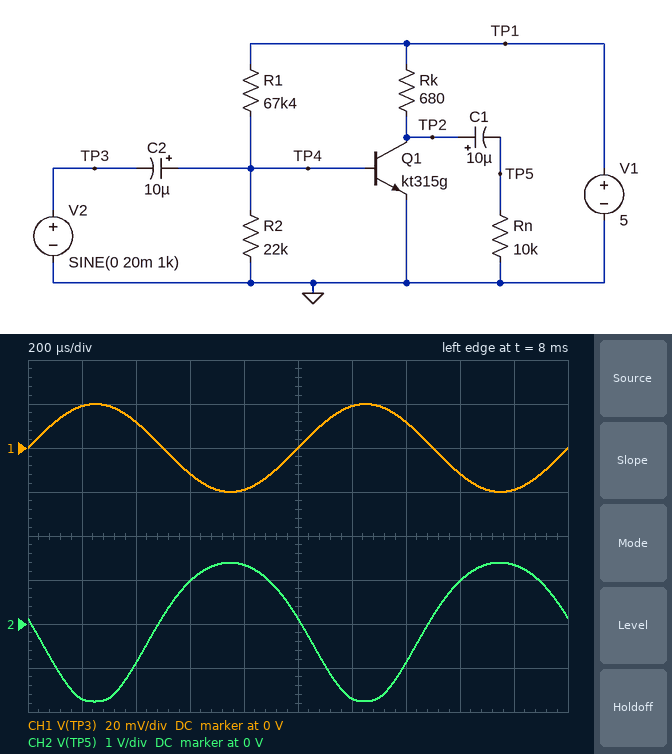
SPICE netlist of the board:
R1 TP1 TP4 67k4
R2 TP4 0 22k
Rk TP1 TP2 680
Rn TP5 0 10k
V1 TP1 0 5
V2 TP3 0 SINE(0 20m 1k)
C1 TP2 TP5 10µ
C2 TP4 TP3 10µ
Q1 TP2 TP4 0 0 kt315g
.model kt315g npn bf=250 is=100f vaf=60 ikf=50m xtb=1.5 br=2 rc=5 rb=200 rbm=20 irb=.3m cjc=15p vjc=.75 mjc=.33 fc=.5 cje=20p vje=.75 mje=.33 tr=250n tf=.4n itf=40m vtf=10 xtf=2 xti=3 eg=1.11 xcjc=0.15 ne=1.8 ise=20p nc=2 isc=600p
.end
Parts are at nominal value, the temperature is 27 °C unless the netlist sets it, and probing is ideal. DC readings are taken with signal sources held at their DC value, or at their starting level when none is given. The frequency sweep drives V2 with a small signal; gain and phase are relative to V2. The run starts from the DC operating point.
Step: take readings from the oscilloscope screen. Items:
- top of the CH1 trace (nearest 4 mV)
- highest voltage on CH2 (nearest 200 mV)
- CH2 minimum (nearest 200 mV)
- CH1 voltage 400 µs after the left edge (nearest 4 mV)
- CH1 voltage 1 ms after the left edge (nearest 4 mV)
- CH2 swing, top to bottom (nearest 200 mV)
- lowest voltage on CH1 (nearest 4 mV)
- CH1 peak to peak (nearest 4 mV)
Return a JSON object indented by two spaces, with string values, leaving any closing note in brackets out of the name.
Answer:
{
  "top of the CH1 trace": "20 mV",
  "highest voltage on CH2": "1.4 V",
  "CH2 minimum": "-1.8 V",
  "CH1 voltage 400 µs after the left edge": "12 mV",
  "CH1 voltage 1 ms after the left edge": "0 V",
  "CH2 swing, top to bottom": "3.2 V",
  "lowest voltage on CH1": "-20 mV",
  "CH1 peak to peak": "40 mV"
}
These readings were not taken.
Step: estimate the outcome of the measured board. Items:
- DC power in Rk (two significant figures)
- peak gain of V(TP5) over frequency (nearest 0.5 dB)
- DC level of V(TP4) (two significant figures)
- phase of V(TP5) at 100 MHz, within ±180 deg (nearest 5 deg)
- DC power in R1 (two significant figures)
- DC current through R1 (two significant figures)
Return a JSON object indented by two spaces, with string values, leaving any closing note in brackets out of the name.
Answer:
{
  "DC power in Rk": "13 mW",
  "peak gain of V(TP5) over frequency": "38.0 dB",
  "DC level of V(TP4)": "640 mV",
  "phase of V(TP5) at 100 MHz, within ±180 deg": "35 deg",
  "DC power in R1": "280 µW",
  "DC current through R1": "65 µA"
}
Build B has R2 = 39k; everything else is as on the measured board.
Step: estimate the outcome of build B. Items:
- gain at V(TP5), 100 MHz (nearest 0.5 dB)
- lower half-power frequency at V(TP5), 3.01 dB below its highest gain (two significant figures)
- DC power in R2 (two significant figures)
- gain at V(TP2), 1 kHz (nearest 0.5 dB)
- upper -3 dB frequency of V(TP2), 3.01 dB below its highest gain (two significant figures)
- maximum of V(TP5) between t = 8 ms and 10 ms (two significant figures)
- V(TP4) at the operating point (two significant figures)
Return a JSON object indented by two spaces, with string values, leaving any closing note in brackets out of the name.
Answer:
{
  "gain at V(TP5), 100 MHz": "7.0 dB",
  "lower half-power frequency at V(TP5), 3.01 dB below its highest gain": "20 Hz",
  "DC power in R2": "11 µW",
  "gain at V(TP2), 1 kHz": "40.0 dB",
  "upper -3 dB frequency of V(TP2), 3.01 dB below its highest gain": "2.8 MHz",
  "maximum of V(TP5) between t = 8 ms and 10 ms": "2.1 V",
  "V(TP4) at the operating point": "650 mV"
}
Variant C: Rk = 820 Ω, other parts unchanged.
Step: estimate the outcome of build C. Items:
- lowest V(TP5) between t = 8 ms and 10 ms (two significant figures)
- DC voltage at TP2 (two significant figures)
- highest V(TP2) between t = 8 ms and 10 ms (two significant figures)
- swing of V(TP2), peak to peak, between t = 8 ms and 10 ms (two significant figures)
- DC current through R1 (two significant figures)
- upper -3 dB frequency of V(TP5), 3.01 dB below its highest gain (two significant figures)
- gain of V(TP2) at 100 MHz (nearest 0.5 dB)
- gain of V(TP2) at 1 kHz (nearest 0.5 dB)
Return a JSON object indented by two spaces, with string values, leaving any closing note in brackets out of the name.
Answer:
{
  "lowest V(TP5) between t = 8 ms and 10 ms": "-1.3 V",
  "DC voltage at TP2": "1.4 V",
  "highest V(TP2) between t = 8 ms and 10 ms": "3.2 V",
  "swing of V(TP2), peak to peak, between t = 8 ms and 10 ms": "3.0 V",
  "DC current through R1": "65 µA",
  "upper -3 dB frequency of V(TP5), 3.01 dB below its highest gain": "3.3 MHz",
  "gain of V(TP2) at 100 MHz": "7.5 dB",
  "gain of V(TP2) at 1 kHz": "39.5 dB"
}
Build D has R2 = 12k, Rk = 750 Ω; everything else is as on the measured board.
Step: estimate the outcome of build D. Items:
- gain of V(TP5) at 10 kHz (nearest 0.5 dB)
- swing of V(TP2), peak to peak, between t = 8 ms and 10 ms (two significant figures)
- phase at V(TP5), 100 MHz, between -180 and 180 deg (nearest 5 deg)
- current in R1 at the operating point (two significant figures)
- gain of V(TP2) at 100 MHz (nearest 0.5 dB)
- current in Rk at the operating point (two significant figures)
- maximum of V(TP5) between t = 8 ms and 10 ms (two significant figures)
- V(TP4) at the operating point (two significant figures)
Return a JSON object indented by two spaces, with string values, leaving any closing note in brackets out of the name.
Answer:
{
  "gain of V(TP5) at 10 kHz": "31.0 dB",
  "swing of V(TP2), peak to peak, between t = 8 ms and 10 ms": "1.5 V",
  "phase at V(TP5), 100 MHz, between -180 and 180 deg": "30 deg",
  "current in R1 at the operating point": "65 µA",
  "gain of V(TP2) at 100 MHz": "6.5 dB",
  "current in Rk at the operating point": "1.5 mA",
  "maximum of V(TP5) between t = 8 ms and 10 ms": "550 mV",
  "V(TP4) at the operating point": "610 mV"
}
